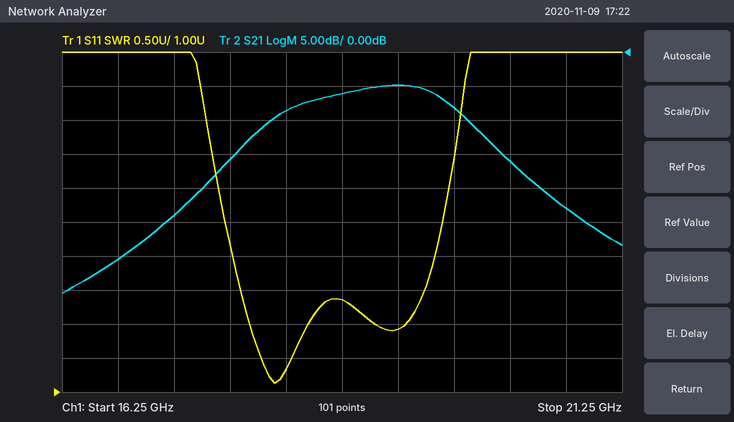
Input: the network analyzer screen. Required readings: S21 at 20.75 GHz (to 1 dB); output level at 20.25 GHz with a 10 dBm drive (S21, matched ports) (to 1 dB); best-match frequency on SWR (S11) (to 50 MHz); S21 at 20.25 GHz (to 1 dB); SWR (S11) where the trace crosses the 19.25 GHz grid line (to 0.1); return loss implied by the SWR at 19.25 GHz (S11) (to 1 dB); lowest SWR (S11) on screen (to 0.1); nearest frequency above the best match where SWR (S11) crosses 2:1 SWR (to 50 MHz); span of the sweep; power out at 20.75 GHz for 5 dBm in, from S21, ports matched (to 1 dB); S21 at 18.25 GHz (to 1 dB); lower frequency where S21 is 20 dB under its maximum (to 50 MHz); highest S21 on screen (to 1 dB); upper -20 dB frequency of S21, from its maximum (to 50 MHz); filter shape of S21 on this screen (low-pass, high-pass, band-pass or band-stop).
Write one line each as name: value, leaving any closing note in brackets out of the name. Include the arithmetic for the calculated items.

S21 at 20.75 GHz: -23 dB
output level at 20.25 GHz with a 10 dBm drive (S21, matched ports): 10 dBm + (-16 dB) = -6 dBm
best-match frequency on SWR (S11): 18.15 GHz
S21 at 20.25 GHz: -16 dB
SWR (S11) where the trace crosses the 19.25 GHz grid line: 1.9
return loss implied by the SWR at 19.25 GHz (S11): −20 log10((1.9 − 1)/(1.9 + 1)) ≈ 10 dB
lowest SWR (S11) on screen: 1.1
nearest frequency above the best match where SWR (S11) crosses 2:1 SWR: 18.45 GHz
span of the sweep: 5 GHz
power out at 20.75 GHz for 5 dBm in, from S21, ports matched: 5 dBm + (-23 dB) = -18 dBm
S21 at 18.25 GHz: -9 dB
lower frequency where S21 is 20 dB under its maximum: 17.20 GHz
highest S21 on screen: -5 dB
upper -20 dB frequency of S21, from its maximum: 20.90 GHz
filter shape of S21 on this screen: band-pass
